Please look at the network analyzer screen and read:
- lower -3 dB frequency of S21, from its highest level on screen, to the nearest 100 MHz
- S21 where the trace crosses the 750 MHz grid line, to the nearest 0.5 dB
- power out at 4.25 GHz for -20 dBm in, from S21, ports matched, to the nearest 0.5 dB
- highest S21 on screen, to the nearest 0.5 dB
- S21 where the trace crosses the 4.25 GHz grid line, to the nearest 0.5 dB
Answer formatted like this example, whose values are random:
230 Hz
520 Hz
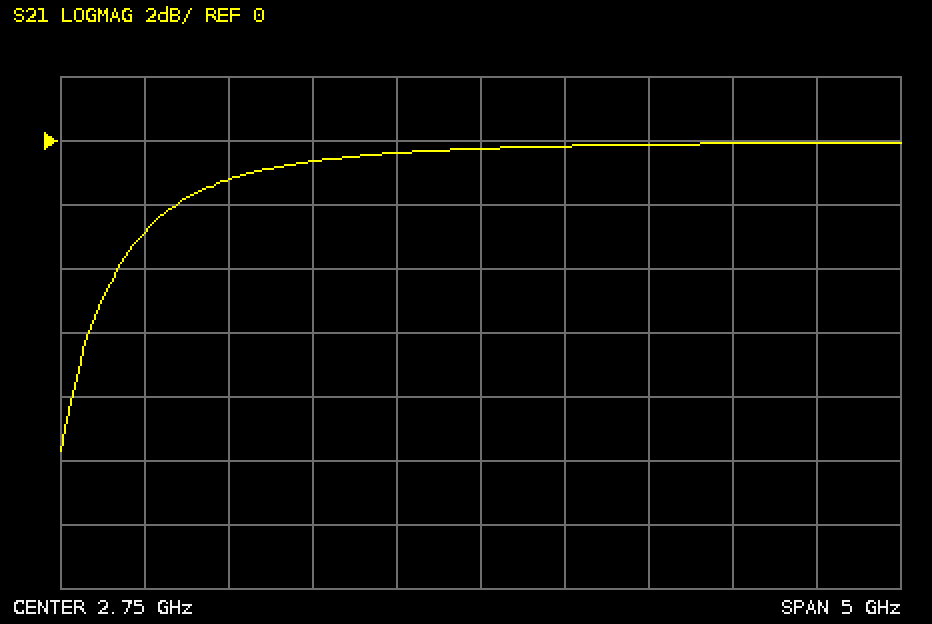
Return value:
700 MHz
-3.0 dB
-20.0 dBm
0.0 dB
0.0 dB
